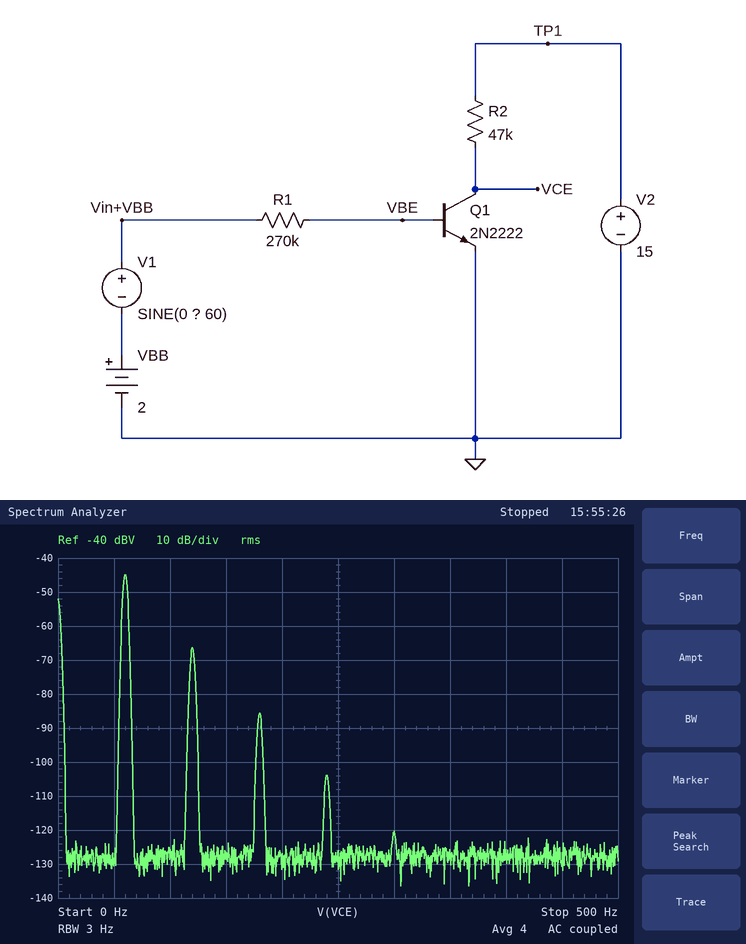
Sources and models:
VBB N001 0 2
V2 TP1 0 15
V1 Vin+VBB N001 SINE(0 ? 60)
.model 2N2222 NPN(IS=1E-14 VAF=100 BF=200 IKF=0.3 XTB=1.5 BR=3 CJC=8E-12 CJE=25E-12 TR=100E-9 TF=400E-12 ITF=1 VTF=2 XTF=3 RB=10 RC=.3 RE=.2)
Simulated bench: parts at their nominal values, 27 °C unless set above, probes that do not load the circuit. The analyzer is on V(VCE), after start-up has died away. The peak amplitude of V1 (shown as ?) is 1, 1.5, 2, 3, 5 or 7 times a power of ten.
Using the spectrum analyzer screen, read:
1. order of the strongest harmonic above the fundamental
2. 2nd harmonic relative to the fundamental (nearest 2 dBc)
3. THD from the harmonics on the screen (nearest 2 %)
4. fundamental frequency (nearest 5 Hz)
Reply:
2
-22 dBc
8 %
60 Hz
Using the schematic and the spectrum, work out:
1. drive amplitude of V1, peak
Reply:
300 mV
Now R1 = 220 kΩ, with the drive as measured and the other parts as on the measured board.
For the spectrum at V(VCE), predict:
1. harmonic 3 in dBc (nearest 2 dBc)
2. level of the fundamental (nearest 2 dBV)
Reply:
-42 dBc
-46 dBV
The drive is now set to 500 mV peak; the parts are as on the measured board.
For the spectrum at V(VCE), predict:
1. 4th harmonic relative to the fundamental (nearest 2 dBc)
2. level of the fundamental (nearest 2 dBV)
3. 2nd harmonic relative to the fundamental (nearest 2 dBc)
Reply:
-44 dBc
-40 dBV
-16 dBc
